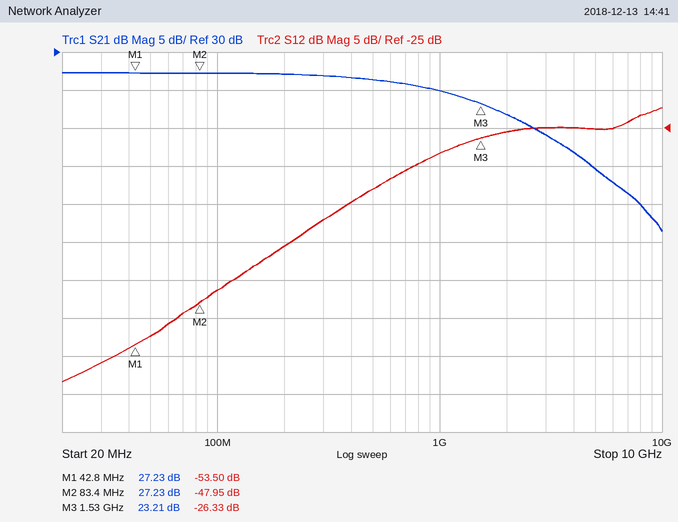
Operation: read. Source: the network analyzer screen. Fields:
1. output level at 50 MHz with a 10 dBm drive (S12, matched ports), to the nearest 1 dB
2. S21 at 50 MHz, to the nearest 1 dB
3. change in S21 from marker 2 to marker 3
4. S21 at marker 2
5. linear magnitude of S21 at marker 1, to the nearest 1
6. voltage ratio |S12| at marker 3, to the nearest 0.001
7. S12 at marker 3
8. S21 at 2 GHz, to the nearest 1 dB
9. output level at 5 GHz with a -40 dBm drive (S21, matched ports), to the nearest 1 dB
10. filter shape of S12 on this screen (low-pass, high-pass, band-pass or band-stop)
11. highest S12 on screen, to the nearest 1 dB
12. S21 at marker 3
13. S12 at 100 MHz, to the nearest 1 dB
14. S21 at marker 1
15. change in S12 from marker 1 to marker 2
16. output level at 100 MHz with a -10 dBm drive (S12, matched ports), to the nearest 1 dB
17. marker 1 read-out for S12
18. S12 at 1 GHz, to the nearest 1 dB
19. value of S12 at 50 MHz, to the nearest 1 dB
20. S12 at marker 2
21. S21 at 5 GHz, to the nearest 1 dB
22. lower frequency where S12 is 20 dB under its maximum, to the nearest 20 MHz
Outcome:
-42 dBm
27 dB
-4.02 dB
27.23 dB
23
0.048
-26.33 dB
22 dB
-25 dBm
high-pass
-22 dB
23.21 dB
-46 dB
27.23 dB
5.55 dB
-56 dBm
-53.50 dB
-28 dB
-52 dB
-47.95 dB
15 dB
160 MHz
